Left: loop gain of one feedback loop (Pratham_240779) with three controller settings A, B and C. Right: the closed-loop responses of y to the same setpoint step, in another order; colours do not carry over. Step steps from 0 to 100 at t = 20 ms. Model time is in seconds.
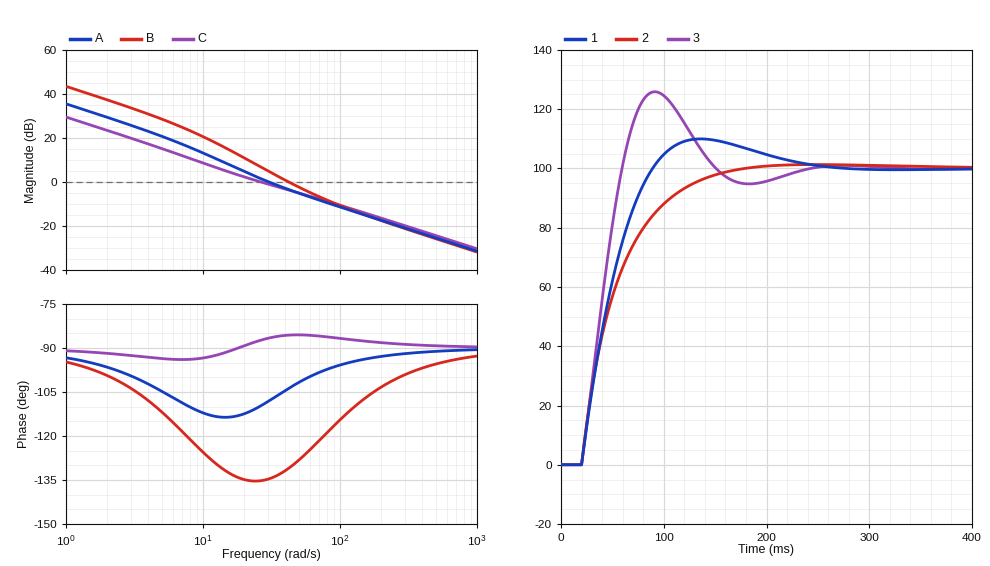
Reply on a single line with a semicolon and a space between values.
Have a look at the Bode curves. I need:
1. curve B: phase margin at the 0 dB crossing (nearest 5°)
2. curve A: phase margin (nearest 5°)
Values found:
50°; 70°
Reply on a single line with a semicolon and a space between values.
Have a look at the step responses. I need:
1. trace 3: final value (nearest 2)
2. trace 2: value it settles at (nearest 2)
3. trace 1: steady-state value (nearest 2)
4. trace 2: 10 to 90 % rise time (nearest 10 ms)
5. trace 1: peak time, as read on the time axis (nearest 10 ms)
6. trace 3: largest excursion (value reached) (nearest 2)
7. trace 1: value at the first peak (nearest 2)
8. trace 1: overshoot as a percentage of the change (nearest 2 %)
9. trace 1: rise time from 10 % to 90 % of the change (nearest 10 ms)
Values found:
100; 100; 100; 80 ms; 140 ms; 126; 110; 10 %; 50 ms
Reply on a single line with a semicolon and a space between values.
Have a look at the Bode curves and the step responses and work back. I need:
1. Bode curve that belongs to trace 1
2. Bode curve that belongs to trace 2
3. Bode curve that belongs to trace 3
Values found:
A; C; B
